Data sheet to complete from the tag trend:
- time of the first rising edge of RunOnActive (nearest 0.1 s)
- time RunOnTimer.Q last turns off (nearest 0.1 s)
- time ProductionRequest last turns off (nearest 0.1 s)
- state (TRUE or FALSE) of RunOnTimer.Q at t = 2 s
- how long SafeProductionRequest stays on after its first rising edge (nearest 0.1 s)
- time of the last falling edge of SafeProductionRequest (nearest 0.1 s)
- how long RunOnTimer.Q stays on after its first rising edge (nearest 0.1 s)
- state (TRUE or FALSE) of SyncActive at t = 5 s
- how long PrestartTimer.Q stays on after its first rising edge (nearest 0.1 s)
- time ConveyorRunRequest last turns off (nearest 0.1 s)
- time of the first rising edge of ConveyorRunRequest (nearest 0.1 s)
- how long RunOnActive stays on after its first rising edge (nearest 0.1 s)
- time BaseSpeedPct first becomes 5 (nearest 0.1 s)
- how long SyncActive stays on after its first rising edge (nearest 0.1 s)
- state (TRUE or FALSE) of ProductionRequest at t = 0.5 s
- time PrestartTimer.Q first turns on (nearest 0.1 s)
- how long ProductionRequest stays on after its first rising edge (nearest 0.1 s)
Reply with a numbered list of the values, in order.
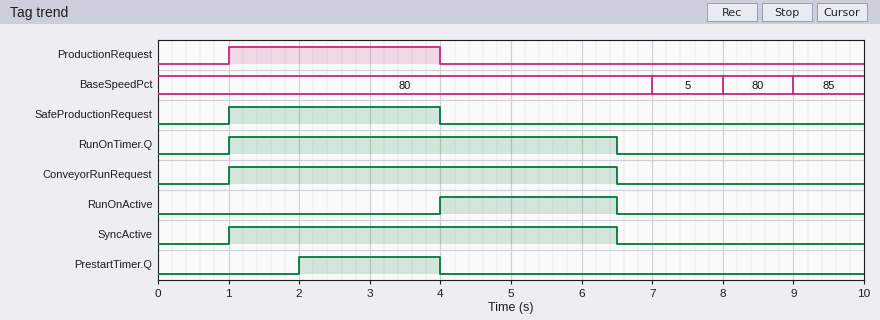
1. 4.0 s
2. 6.5 s
3. 4.0 s
4. TRUE
5. 3.0 s
6. 4.0 s
7. 5.5 s
8. TRUE
9. 2.0 s
10. 6.5 s
11. 1.0 s
12. 2.5 s
13. 7.0 s
14. 5.5 s
15. FALSE
16. 2.0 s
17. 3.0 s
